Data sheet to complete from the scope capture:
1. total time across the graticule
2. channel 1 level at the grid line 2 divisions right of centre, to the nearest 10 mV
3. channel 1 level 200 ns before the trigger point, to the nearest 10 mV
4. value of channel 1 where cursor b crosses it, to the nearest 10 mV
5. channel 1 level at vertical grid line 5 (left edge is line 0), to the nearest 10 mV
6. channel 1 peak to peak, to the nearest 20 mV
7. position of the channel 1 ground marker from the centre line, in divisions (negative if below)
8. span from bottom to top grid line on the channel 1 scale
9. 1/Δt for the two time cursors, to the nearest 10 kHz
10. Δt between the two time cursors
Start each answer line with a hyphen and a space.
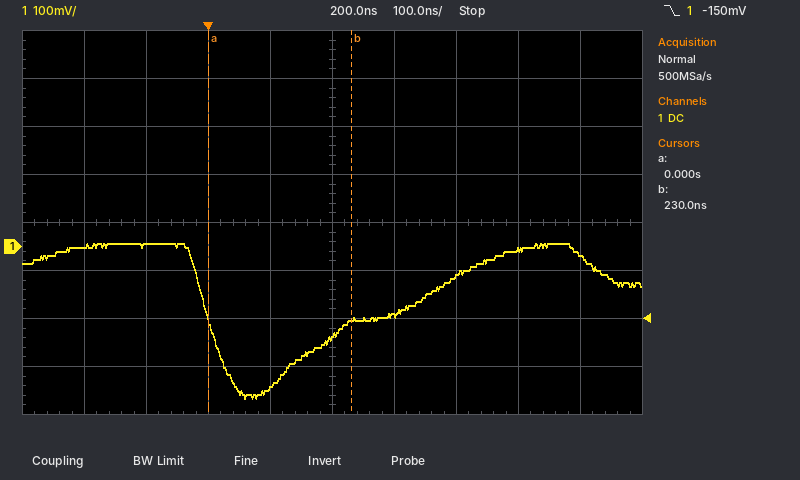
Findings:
- 1 µs
- -60 mV
- 0 mV
- -150 mV
- -190 mV
- 320 mV
- -0.5 div
- 800 mV
- 4.35 MHz
- 230 ns
